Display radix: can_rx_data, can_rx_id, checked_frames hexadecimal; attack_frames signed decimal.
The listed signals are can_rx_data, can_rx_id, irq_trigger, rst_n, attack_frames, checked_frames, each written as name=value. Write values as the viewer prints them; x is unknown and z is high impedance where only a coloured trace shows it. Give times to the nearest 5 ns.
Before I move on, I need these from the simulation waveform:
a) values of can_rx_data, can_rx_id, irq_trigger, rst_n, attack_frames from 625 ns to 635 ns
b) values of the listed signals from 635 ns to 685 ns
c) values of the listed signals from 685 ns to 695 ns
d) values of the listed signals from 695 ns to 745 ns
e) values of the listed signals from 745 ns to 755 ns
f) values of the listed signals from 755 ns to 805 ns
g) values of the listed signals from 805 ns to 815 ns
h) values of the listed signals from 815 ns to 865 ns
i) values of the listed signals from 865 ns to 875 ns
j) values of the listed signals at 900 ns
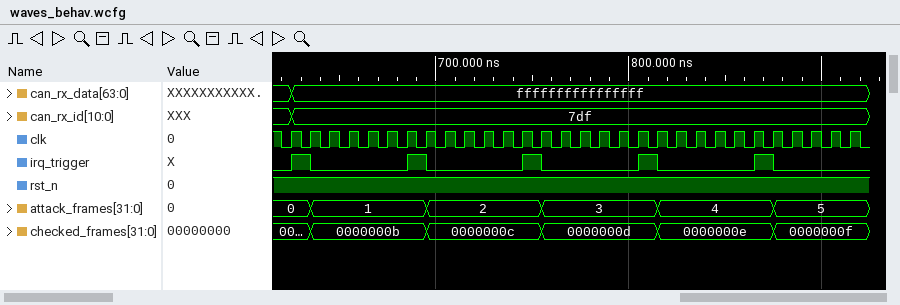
can_rx_data=ffffffffffffffff, can_rx_id=7df, irq_trigger=1, rst_n=1, attack_frames=0
can_rx_data=ffffffffffffffff, can_rx_id=7df, irq_trigger=0, rst_n=1, attack_frames=1, checked_frames=0000000b
can_rx_data=ffffffffffffffff, can_rx_id=7df, irq_trigger=1, rst_n=1, attack_frames=1, checked_frames=0000000b
can_rx_data=ffffffffffffffff, can_rx_id=7df, irq_trigger=0, rst_n=1, attack_frames=2, checked_frames=0000000c
can_rx_data=ffffffffffffffff, can_rx_id=7df, irq_trigger=1, rst_n=1, attack_frames=2, checked_frames=0000000c
can_rx_data=ffffffffffffffff, can_rx_id=7df, irq_trigger=0, rst_n=1, attack_frames=3, checked_frames=0000000d
can_rx_data=ffffffffffffffff, can_rx_id=7df, irq_trigger=1, rst_n=1, attack_frames=3, checked_frames=0000000d
can_rx_data=ffffffffffffffff, can_rx_id=7df, irq_trigger=0, rst_n=1, attack_frames=4, checked_frames=0000000e
can_rx_data=ffffffffffffffff, can_rx_id=7df, irq_trigger=1, rst_n=1, attack_frames=4, checked_frames=0000000e
can_rx_data=ffffffffffffffff, can_rx_id=7df, irq_trigger=0, rst_n=1, attack_frames=5, checked_frames=0000000f
